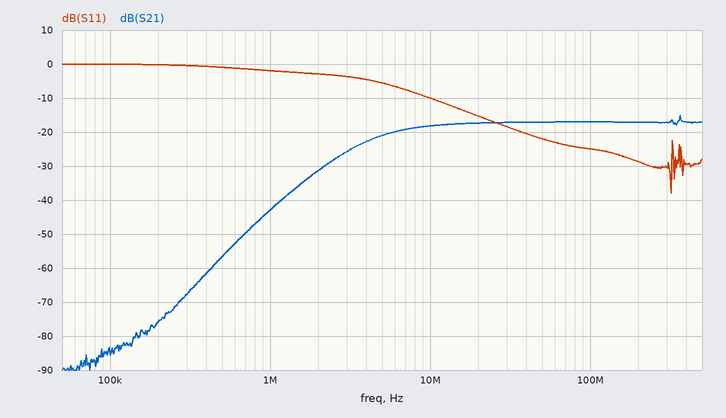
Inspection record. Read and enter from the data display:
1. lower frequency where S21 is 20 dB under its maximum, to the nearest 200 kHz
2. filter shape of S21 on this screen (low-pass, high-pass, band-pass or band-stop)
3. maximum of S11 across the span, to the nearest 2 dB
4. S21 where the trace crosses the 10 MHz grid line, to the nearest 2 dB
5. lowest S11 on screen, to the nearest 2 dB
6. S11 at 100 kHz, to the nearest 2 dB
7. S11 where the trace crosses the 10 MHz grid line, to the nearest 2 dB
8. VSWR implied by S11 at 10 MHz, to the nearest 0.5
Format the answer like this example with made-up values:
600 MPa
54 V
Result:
1.6 MHz
high-pass
0 dB
-18 dB
-38 dB
0 dB
-10 dB
2.0
